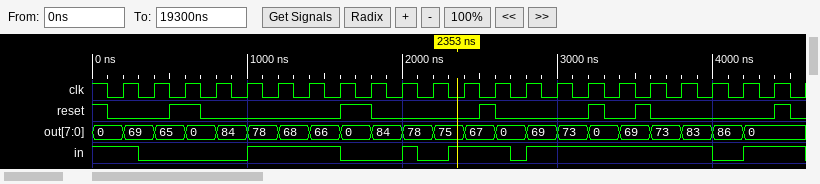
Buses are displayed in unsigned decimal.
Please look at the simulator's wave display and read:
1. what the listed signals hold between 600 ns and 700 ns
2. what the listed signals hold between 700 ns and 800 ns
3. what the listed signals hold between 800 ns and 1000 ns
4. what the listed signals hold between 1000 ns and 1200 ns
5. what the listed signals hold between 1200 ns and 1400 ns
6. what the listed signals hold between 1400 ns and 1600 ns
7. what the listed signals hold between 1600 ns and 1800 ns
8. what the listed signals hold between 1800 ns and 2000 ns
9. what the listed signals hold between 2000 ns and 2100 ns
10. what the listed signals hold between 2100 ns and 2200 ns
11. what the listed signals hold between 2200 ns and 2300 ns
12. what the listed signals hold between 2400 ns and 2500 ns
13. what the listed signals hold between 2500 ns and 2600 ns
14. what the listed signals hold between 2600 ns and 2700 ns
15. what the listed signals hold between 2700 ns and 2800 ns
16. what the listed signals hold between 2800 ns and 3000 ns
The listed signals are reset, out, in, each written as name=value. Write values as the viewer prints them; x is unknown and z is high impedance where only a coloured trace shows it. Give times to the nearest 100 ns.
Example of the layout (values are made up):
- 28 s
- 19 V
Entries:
- reset=1, out=0, in=0
- reset=0, out=0, in=0
- reset=0, out=84, in=0
- reset=0, out=78, in=1
- reset=0, out=68, in=1
- reset=0, out=66, in=1
- reset=1, out=0, in=0
- reset=0, out=84, in=0
- reset=0, out=78, in=1
- reset=0, out=78, in=0
- reset=0, out=75, in=0
- reset=0, out=67, in=1
- reset=1, out=67, in=1
- reset=0, out=0, in=1
- reset=0, out=0, in=0
- reset=0, out=69, in=1
